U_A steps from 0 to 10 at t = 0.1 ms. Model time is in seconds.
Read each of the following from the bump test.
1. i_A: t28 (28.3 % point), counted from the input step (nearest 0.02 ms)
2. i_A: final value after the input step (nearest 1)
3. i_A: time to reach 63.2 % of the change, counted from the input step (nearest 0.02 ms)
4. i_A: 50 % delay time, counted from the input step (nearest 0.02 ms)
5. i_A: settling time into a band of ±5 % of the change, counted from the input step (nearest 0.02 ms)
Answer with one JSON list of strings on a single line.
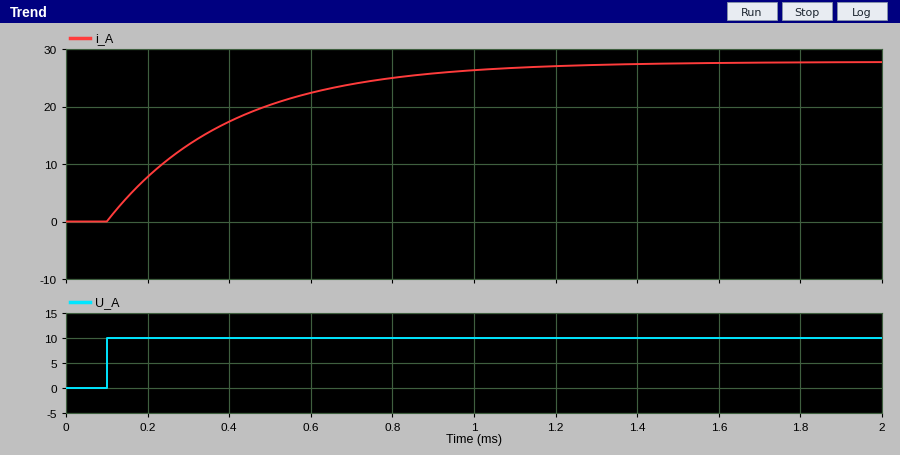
["0.10 ms", "28", "0.30 ms", "0.22 ms", "0.92 ms"]
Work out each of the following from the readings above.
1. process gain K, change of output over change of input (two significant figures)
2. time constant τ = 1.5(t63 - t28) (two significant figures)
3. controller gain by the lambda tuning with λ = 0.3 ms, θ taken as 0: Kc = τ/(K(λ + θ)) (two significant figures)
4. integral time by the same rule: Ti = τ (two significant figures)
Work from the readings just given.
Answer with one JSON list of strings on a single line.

["2.8", "0.30 ms", "0.36", "0.30 ms"]
